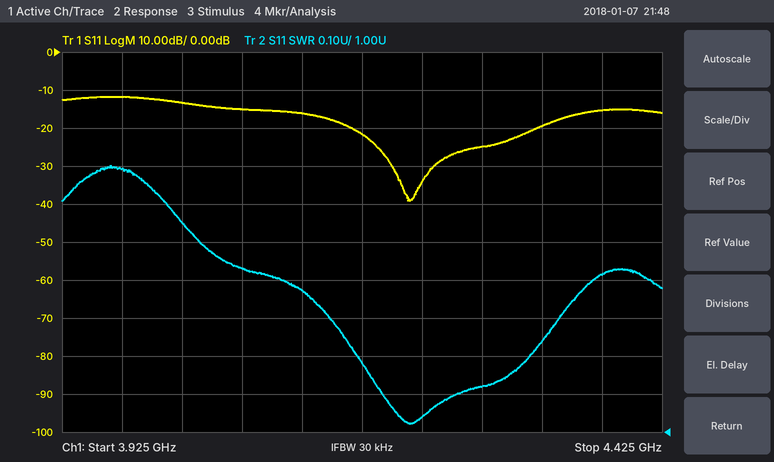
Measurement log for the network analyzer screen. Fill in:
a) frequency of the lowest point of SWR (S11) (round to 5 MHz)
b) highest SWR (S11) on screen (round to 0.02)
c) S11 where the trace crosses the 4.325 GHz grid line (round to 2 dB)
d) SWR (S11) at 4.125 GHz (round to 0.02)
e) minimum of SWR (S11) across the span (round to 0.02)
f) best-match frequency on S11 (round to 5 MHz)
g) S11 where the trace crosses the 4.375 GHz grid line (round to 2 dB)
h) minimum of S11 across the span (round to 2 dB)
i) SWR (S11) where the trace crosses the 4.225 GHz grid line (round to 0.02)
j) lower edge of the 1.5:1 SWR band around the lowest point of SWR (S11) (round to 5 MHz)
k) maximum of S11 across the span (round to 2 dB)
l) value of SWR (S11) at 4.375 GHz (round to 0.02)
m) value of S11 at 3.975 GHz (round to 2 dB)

4.215 GHz
1.70
-20 dB
1.38
1.02
4.215 GHz
-16 dB
-40 dB
1.04
4.040 GHz
-12 dB
1.42
-12 dB
